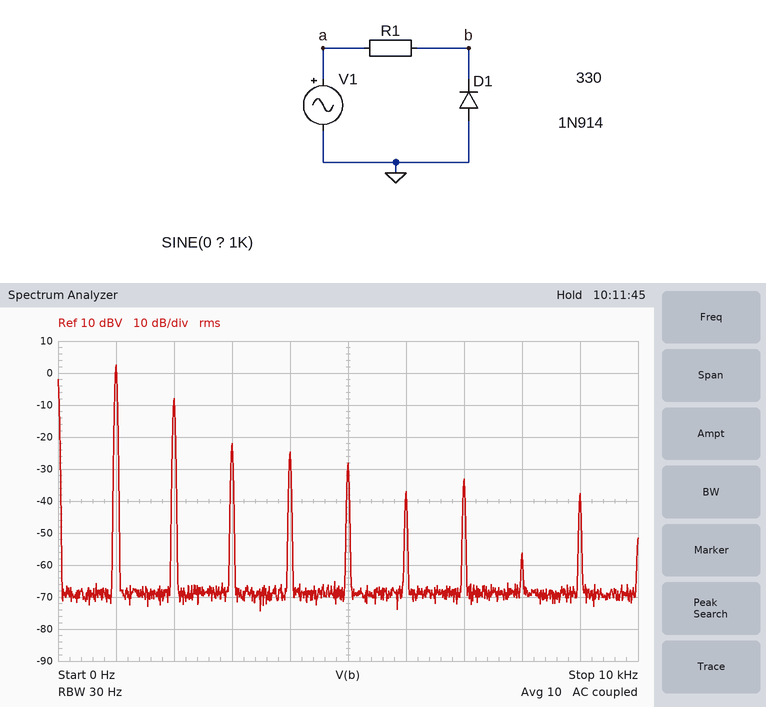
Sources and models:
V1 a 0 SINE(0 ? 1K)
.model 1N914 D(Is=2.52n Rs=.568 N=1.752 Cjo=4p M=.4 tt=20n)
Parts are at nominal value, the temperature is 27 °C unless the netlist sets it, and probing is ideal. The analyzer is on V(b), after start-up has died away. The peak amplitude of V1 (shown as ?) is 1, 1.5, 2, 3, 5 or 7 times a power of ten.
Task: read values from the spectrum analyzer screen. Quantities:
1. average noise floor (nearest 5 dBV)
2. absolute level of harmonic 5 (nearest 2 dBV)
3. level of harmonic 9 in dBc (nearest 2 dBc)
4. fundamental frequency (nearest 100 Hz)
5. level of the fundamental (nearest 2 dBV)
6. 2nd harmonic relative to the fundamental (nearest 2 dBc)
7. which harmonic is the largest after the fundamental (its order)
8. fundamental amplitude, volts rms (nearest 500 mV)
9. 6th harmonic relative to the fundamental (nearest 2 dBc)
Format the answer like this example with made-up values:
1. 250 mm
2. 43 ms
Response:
1. -70 dBV
2. -28 dBV
3. -40 dBc
4. 1.0 kHz
5. 2 dBV
6. -10 dBc
7. 2
8. 1.5 V
9. -40 dBc
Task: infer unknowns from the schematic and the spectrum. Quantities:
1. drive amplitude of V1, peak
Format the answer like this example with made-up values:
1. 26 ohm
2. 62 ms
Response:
1. 3 V
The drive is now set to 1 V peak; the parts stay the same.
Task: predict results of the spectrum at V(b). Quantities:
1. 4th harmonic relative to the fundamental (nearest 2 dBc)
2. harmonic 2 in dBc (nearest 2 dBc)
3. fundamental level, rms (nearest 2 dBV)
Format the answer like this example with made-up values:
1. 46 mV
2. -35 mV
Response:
1. -36 dBc
2. -18 dBc
3. -4 dBV
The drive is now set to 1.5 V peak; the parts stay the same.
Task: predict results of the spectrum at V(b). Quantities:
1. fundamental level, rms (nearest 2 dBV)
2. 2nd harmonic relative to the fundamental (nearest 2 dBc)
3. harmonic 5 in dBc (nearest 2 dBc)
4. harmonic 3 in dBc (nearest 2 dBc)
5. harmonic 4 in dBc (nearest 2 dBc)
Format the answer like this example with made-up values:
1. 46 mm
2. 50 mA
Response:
1. -2 dBV
2. -14 dBc
3. -32 dBc
4. -22 dBc
5. -44 dBc
